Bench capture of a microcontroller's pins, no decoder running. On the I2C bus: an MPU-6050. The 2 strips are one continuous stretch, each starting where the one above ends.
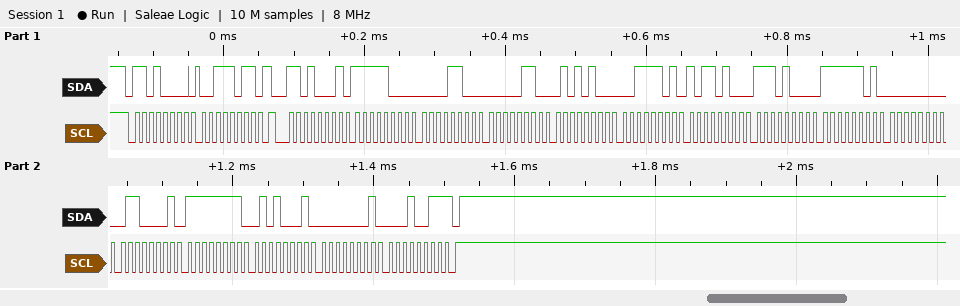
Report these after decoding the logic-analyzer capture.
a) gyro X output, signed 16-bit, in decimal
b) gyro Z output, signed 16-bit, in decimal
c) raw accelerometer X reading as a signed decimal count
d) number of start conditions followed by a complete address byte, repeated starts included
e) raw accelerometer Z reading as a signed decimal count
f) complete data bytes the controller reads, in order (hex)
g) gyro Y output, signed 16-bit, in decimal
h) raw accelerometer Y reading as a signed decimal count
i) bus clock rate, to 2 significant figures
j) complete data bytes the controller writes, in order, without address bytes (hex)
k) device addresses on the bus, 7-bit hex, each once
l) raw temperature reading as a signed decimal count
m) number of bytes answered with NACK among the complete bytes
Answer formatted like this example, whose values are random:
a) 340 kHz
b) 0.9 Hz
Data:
a) 97
b) 275
c) -2036
d) 2
e) 15796
f) F8 0C 06 54 3D B4 E8 FD 00 61 FF 51 01 13
g) -175
h) 1620
i) 100 kHz
j) 3B
k) 0x68
l) -5891
m) 1
